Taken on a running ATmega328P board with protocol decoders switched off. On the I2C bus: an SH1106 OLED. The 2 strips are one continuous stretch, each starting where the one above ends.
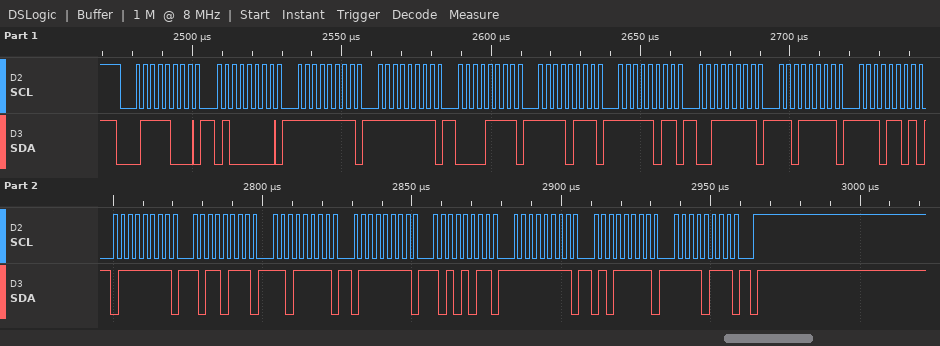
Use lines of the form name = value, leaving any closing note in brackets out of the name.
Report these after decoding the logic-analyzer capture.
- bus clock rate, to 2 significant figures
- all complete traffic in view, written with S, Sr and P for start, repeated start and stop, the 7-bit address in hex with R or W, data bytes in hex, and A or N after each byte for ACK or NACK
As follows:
bus clock rate, to 2 significant figures = 400 kHz
all complete traffic in view, written with S, Sr and P for start, repeated start and stop, the 7-bit address in hex with R or W, data bytes in hex, and A or N after each byte for ACK or NACK = S 3CW A 40 A FF A FF A 0F A F7 A FB A 3F A DF A ED A 7F A B7 A DF A 7F A AB A FF A 5F A F7 A P
